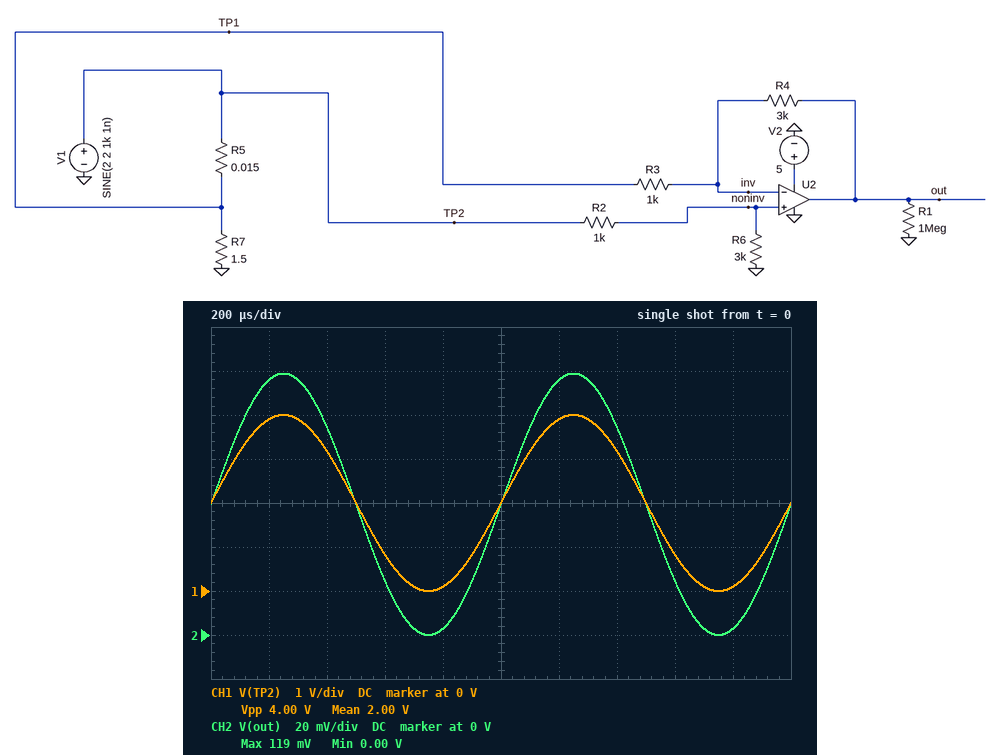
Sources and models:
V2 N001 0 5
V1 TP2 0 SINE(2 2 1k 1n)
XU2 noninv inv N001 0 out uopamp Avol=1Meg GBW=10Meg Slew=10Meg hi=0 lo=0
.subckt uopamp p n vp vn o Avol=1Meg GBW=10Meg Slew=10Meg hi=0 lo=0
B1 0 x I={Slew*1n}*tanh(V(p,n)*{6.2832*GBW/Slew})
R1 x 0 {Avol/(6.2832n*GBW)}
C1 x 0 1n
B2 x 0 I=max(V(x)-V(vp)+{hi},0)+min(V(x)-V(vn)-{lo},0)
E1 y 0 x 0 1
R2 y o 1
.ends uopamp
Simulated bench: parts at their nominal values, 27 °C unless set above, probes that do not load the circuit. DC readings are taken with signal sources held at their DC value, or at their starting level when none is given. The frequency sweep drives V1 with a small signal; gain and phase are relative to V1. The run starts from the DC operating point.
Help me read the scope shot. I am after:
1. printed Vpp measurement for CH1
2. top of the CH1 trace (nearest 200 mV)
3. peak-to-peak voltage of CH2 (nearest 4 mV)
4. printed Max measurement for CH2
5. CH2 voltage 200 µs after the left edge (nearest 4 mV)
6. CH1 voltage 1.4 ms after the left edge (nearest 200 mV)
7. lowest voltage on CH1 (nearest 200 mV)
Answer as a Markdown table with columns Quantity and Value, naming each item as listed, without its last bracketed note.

| Quantity | Value |
|---|---|
| printed Vpp measurement for CH1 | 4.00 V |
| top of the CH1 trace | 4.0 V |
| peak-to-peak voltage of CH2 | 120 mV |
| printed Max measurement for CH2 | 119 mV |
| CH2 voltage 200 µs after the left edge | 116 mV |
| CH1 voltage 1.4 ms after the left edge | 3.2 V |
| lowest voltage on CH1 | 0 V |
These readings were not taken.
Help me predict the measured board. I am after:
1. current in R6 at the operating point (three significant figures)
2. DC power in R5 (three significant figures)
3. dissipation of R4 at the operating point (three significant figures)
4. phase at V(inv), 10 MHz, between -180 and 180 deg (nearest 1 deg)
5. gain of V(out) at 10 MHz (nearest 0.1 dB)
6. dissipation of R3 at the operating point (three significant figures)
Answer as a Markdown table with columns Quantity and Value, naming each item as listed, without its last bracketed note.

| Quantity | Value |
|---|---|
| current in R6 at the operating point | 500 µA |
| DC power in R5 | 26.2 mW |
| dissipation of R4 at the operating point | 692 µW |
| phase at V(inv), 10 MHz, between -180 and 180 deg | 0 deg |
| gain of V(out) at 10 MHz | -42.8 dB |
| dissipation of R3 at the operating point | 231 µW |
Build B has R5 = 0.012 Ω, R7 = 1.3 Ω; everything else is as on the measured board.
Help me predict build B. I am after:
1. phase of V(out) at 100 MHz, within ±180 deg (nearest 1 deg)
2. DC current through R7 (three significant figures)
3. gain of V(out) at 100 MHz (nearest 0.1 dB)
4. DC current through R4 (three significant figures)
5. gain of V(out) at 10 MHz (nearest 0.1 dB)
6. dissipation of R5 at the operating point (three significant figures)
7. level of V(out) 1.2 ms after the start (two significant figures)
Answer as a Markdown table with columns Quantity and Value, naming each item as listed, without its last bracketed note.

| Quantity | Value |
|---|---|
| phase of V(out) at 100 MHz, within ±180 deg | -69 deg |
| DC current through R7 | 1.52 A |
| gain of V(out) at 100 MHz | -62.7 dB |
| DC current through R4 | 482 µA |
| gain of V(out) at 10 MHz | -43.5 dB |
| dissipation of R5 at the operating point | 27.9 mW |
| level of V(out) 1.2 ms after the start | 110 mV |
